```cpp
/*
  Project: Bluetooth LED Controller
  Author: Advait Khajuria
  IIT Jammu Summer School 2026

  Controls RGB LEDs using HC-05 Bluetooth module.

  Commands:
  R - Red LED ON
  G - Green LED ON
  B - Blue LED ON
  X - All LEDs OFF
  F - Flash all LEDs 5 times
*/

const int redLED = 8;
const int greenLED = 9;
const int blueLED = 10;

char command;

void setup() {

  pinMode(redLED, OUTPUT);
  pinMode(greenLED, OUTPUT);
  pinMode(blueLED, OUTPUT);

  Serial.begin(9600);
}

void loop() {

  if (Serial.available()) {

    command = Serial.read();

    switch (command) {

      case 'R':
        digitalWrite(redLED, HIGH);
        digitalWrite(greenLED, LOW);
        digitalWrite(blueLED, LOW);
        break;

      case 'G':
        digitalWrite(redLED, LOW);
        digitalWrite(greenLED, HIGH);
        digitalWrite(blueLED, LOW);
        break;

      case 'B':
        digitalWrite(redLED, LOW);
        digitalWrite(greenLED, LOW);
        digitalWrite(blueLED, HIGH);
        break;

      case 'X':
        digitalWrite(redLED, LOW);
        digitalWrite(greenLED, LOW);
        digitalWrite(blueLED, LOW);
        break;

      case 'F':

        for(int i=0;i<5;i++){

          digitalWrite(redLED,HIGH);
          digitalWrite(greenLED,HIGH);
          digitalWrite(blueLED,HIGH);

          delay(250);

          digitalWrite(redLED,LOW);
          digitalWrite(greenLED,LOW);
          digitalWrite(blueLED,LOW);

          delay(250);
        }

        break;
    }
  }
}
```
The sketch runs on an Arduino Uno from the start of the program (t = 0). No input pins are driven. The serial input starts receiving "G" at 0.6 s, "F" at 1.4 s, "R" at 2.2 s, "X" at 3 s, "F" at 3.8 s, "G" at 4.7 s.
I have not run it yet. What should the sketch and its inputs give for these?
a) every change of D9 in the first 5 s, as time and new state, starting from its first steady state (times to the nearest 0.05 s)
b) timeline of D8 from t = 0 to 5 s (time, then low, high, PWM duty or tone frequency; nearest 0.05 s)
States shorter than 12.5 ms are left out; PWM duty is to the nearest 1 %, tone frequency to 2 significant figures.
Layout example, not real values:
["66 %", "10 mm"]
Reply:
["0 s low; 0.6 s high; 1.65 s low; 1.9 s high; 2.15 s low; 2.4 s high; 2.65 s low; 2.9 s high; 3.15 s low; 3.4 s high; 3.65 s low; 3.9 s high; 4.15 s low; 4.4 s high; 4.65 s low; 4.9 s high", "0 s low; 1.4 s high; 1.65 s low; 1.9 s high; 2.15 s low; 2.4 s high; 2.65 s low; 2.9 s high; 3.15 s low; 3.4 s high; 3.65 s low; 3.9 s high; 4.15 s low; 4.4 s high; 4.65 s low; 4.9 s high"]
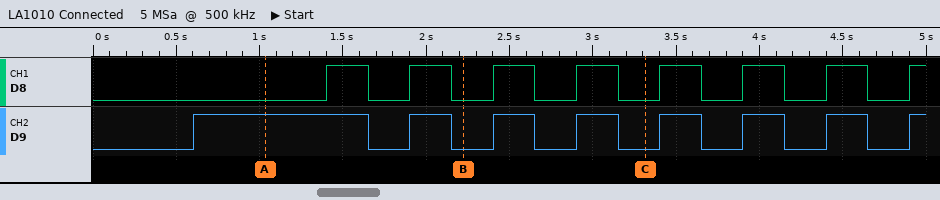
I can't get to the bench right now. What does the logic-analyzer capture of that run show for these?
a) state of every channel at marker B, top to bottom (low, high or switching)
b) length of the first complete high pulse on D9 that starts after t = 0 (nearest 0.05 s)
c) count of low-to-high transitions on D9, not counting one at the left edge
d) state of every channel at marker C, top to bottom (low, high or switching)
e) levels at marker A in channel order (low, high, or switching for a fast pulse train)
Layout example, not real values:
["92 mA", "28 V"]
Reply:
["D8 low, D9 low", "1.05 s", "8", "D8 low, D9 low", "D8 low, D9 high"]
